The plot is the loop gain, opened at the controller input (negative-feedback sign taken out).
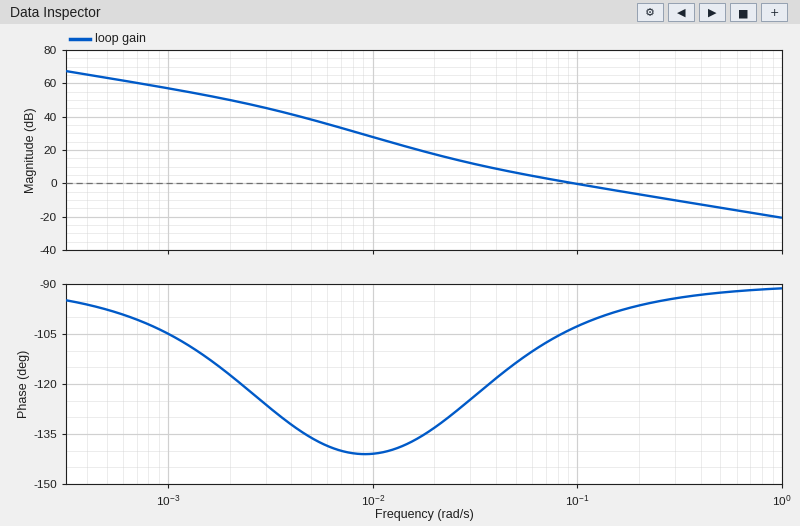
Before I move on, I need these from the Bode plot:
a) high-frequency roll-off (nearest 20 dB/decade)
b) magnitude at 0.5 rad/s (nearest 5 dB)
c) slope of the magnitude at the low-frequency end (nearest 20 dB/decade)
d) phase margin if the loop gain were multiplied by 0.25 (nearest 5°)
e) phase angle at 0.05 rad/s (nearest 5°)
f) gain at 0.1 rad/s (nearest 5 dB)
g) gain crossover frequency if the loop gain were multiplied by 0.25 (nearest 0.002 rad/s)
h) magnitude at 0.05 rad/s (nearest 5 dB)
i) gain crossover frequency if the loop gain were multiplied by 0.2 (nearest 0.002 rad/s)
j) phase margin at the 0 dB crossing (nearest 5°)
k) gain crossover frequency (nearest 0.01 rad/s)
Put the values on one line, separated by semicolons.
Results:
-20 dB/decade; -15 dB; -20 dB/decade; 55°; -115°; 0 dB; 0.030 rad/s; 5 dB; 0.026 rad/s; 75°; 0.10 rad/s
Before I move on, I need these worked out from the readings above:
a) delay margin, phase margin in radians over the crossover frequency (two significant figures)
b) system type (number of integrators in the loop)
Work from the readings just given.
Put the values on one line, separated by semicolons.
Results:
13 s; 1
